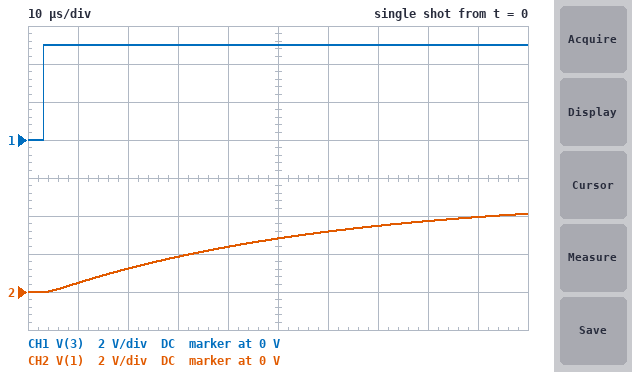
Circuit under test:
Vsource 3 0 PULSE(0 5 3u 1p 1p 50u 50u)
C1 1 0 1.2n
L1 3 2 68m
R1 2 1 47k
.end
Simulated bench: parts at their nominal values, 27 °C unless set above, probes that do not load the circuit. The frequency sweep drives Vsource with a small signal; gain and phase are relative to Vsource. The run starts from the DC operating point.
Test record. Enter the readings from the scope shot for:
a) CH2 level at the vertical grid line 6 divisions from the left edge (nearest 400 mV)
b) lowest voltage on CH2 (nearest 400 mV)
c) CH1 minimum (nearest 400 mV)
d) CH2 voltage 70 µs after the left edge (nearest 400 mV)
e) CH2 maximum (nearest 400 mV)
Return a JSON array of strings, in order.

["3.2 V", "0 V", "0 V", "3.6 V", "4.0 V"]
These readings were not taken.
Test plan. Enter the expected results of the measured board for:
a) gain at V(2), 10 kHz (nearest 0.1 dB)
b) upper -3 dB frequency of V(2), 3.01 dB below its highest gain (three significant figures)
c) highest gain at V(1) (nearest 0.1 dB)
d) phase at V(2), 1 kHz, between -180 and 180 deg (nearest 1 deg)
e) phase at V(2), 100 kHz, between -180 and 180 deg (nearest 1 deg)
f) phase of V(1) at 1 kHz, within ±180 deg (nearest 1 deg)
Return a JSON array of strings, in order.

["0.2 dB", "108 kHz", "0 dB", "0 deg", "-43 deg", "-20 deg"]
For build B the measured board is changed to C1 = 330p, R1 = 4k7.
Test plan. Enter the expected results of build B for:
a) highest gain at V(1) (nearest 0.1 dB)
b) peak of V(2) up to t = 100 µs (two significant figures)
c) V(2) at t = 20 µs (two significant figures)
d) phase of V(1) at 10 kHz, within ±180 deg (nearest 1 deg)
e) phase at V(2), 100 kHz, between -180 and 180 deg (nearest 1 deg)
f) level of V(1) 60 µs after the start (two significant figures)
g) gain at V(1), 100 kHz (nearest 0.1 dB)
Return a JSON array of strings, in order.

["9.8 dB", "8.1 V", "7.4 V", "-6 deg", "-129 deg", "4.5 V", "-18.0 dB"]
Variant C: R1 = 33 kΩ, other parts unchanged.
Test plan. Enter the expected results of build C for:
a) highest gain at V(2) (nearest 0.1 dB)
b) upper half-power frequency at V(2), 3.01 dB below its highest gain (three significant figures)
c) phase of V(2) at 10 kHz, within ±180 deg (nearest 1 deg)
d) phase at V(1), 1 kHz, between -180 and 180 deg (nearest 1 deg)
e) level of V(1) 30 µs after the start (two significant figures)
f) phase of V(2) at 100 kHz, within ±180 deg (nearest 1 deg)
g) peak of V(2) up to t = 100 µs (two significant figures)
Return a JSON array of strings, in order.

["0.3 dB", "75.5 kHz", "-7 deg", "-14 deg", "2.4 V", "-54 deg", "5.2 V"]
